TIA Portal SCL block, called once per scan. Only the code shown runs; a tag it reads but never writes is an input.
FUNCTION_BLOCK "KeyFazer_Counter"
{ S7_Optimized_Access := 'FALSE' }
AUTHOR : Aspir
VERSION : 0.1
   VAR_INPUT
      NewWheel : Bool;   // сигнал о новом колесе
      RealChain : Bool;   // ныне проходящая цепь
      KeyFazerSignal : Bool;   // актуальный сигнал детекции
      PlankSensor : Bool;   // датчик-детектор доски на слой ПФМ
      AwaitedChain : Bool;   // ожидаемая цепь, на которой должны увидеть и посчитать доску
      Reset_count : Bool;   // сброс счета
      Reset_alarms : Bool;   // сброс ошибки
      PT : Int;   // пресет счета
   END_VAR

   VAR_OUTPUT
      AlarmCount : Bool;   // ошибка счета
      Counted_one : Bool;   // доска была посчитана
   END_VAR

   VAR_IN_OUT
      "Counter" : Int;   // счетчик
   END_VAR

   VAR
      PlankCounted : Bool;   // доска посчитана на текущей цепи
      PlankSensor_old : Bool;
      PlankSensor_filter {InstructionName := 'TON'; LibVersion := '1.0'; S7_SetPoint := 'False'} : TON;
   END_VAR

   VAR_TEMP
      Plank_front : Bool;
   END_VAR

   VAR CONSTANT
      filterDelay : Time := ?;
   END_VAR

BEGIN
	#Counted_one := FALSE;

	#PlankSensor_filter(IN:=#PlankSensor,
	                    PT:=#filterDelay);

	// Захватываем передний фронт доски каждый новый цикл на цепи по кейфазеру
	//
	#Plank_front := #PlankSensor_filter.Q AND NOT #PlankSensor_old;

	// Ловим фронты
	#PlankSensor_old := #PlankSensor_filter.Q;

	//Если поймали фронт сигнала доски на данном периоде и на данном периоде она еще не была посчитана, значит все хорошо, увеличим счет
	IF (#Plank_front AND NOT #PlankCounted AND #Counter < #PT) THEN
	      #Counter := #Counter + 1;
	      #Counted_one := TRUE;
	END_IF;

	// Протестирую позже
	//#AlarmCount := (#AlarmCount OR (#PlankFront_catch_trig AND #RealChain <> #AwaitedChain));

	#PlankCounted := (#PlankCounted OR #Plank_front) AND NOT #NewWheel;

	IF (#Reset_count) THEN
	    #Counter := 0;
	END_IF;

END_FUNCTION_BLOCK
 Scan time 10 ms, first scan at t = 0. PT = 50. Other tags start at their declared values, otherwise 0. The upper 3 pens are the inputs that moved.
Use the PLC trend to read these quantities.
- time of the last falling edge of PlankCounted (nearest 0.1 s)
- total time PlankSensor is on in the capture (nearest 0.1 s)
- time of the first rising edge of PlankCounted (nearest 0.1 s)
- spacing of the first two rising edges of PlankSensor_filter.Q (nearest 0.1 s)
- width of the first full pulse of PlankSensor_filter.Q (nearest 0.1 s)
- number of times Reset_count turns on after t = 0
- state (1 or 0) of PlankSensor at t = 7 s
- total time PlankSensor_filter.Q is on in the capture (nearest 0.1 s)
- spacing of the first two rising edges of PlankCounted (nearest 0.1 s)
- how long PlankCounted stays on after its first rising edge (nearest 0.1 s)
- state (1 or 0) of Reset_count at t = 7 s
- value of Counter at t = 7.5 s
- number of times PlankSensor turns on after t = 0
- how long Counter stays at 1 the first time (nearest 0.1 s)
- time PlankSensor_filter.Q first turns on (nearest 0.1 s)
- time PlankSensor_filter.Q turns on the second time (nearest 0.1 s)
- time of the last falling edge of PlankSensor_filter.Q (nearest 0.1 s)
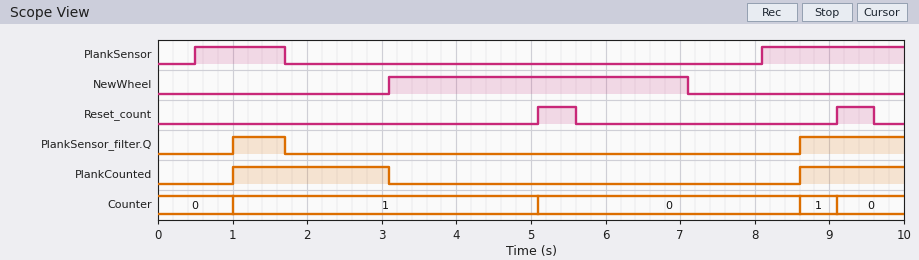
3.1 s
3.1 s
1.0 s
7.6 s
0.7 s
2
0
2.1 s
7.6 s
2.1 s
0
0
2
4.1 s
1.0 s
8.6 s
1.7 s
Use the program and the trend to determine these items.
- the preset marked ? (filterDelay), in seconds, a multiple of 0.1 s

0.5 s
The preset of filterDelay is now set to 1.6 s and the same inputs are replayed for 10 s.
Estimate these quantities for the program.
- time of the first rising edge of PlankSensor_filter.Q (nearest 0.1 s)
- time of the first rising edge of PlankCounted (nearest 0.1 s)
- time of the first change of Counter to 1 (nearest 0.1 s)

9.7 s
9.7 s
9.7 s
